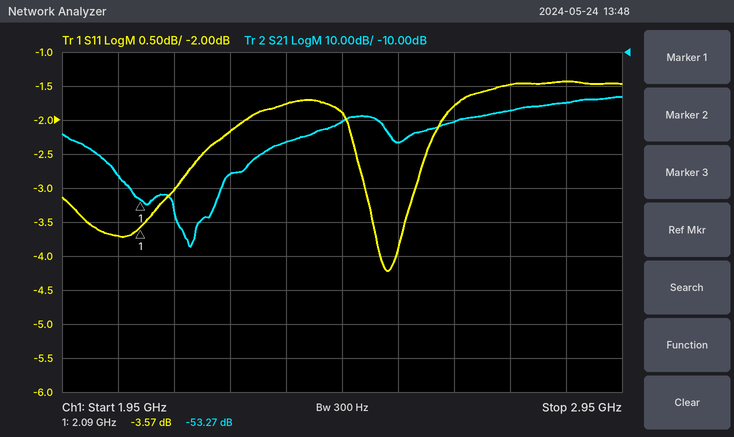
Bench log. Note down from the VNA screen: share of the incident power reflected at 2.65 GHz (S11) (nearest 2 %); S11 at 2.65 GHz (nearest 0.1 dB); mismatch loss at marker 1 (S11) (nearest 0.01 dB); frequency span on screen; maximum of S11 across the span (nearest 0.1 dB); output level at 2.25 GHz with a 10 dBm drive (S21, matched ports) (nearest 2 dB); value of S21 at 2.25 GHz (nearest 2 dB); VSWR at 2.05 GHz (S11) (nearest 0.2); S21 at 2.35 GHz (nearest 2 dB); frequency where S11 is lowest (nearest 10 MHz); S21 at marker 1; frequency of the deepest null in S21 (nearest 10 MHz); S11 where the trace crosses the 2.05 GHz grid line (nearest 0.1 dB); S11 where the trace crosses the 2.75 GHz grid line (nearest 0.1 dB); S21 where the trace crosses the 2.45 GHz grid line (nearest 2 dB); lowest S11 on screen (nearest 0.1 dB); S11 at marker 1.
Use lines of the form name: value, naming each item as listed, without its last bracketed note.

share of the incident power reflected at 2.65 GHz (S11): 66 %
S11 at 2.65 GHz: -1.8 dB
mismatch loss at marker 1 (S11): 2.51 dB
frequency span on screen: 1 GHz
maximum of S11 across the span: -1.4 dB
output level at 2.25 GHz with a 10 dBm drive (S21, matched ports): -36 dBm
value of S21 at 2.25 GHz: -46 dB
VSWR at 2.05 GHz (S11): 4.8
S21 at 2.35 GHz: -36 dB
frequency where S11 is lowest: 2.53 GHz
S21 at marker 1: -53.27 dB
frequency of the deepest null in S21: 2.18 GHz
S11 where the trace crosses the 2.05 GHz grid line: -3.7 dB
S11 where the trace crosses the 2.75 GHz grid line: -1.5 dB
S21 where the trace crosses the 2.45 GHz grid line: -30 dB
lowest S11 on screen: -4.2 dB
S11 at marker 1: -3.57 dB
